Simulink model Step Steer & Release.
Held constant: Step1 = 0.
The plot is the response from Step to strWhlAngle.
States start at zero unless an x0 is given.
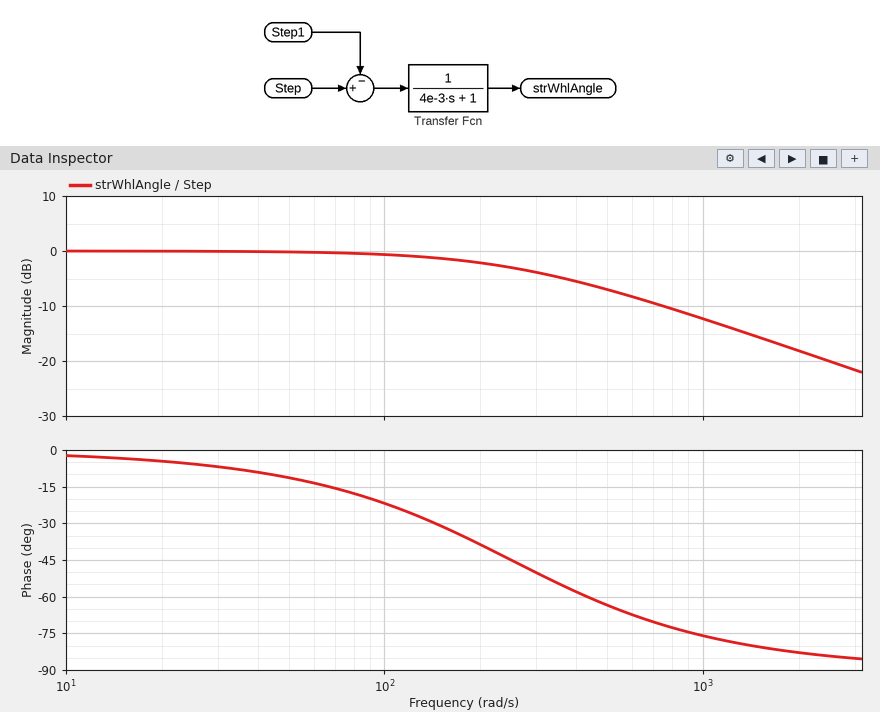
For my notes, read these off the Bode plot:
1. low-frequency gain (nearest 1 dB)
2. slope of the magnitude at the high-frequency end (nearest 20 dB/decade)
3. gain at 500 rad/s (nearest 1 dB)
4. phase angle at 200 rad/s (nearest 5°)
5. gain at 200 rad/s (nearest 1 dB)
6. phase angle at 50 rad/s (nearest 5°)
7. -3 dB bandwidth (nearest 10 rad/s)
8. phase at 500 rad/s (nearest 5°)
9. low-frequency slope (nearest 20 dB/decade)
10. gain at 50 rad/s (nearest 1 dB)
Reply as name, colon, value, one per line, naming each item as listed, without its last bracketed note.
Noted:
low-frequency gain: 0 dB
slope of the magnitude at the high-frequency end: -20 dB/decade
gain at 500 rad/s: -7 dB
phase angle at 200 rad/s: -40°
gain at 200 rad/s: -2 dB
phase angle at 50 rad/s: -10°
-3 dB bandwidth: 250 rad/s
phase at 500 rad/s: -65°
low-frequency slope: 0 dB/decade
gain at 50 rad/s: 0 dB
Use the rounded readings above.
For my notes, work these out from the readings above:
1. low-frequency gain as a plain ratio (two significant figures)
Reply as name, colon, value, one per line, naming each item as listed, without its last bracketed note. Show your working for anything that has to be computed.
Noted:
low-frequency gain as a plain ratio: 10^(0 / 20) = 1.0
